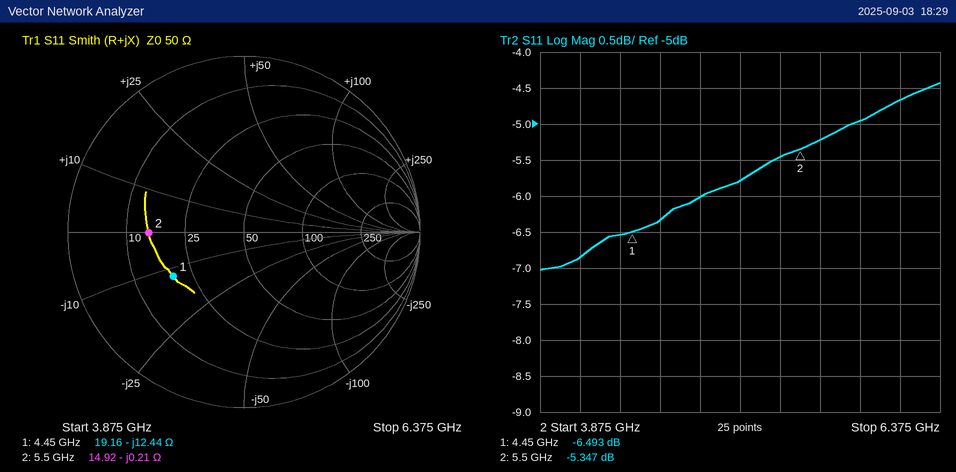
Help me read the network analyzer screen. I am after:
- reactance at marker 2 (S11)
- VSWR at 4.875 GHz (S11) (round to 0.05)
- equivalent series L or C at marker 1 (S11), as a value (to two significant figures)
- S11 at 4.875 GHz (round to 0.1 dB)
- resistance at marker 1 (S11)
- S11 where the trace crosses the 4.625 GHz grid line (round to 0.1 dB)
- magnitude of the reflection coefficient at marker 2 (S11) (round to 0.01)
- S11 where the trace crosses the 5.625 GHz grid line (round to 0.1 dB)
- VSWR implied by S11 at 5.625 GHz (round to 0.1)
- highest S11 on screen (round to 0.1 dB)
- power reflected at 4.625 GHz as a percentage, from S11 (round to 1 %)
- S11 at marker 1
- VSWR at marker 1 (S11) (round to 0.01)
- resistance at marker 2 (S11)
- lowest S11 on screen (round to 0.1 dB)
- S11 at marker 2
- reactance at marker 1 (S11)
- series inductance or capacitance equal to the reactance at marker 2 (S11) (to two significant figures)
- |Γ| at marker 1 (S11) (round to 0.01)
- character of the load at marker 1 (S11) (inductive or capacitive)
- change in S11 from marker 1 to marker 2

-0.21 Ω
3.00
2.9 pF
-6.0 dB
19.16 Ω
-6.3 dB
0.54
-5.2 dB
3.4
-4.4 dB
23 %
-6.493 dB
2.80
14.92 Ω
-7.0 dB
-5.347 dB
-12.44 Ω
140 pF
0.47
capacitive
1.146 dB
